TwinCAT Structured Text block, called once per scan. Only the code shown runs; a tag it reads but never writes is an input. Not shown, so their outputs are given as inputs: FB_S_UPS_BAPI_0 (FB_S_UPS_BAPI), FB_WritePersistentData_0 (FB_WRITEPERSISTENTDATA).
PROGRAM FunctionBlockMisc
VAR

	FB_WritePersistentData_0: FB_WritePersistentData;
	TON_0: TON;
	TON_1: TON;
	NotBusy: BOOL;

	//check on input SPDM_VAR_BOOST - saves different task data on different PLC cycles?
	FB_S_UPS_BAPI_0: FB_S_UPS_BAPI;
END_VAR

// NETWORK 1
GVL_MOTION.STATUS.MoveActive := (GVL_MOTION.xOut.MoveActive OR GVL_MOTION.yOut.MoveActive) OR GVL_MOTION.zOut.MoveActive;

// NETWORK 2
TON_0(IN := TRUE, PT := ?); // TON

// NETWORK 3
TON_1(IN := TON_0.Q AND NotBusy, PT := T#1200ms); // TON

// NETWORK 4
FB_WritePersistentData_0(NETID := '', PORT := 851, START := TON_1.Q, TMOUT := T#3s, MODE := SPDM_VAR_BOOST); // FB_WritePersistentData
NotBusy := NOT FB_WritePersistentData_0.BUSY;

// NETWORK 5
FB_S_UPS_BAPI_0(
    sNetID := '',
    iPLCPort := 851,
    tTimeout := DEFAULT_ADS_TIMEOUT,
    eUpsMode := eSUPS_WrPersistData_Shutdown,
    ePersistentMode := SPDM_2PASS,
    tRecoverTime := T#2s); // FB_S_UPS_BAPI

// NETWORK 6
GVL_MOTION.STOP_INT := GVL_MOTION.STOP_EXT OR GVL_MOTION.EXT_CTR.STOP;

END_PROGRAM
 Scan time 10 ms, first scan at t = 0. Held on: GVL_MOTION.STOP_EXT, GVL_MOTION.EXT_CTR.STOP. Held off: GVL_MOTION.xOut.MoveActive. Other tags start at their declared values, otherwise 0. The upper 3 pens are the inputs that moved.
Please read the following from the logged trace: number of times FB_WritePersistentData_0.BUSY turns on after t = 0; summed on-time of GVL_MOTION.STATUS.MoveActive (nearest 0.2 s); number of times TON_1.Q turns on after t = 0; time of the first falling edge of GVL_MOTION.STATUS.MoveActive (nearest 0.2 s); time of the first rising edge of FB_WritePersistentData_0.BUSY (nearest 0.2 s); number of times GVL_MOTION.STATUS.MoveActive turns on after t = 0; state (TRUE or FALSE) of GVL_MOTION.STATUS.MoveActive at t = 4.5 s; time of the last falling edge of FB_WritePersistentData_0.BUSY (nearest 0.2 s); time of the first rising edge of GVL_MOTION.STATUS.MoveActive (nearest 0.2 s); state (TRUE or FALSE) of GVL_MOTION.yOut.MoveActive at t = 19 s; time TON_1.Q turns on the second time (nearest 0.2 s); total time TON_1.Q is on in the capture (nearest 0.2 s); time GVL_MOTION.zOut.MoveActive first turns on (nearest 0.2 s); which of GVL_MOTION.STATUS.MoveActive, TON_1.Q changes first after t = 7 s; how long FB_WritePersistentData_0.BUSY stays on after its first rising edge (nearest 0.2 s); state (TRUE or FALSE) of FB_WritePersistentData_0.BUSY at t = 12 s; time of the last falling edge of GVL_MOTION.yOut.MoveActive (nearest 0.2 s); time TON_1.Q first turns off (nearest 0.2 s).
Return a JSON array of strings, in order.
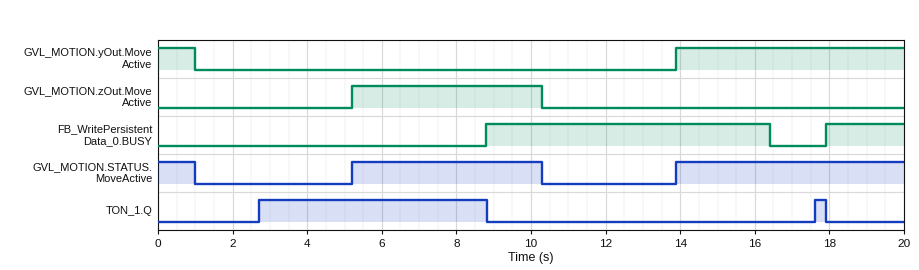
["2", "12.2 s", "2", "1.0 s", "8.8 s", "2", "FALSE", "16.4 s", "5.2 s", "TRUE", "17.6 s", "6.4 s", "5.2 s", "TON_1.Q", "7.6 s", "TRUE", "1.0 s", "8.8 s"]
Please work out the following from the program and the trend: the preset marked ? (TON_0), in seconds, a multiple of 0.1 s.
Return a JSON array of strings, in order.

["1.5 s"]
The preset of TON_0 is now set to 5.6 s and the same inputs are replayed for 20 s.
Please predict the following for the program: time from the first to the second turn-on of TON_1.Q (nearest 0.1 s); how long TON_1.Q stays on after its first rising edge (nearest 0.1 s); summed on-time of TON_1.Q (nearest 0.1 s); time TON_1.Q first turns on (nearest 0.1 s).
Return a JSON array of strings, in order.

["10.8 s", "2.0 s", "2.3 s", "6.8 s"]
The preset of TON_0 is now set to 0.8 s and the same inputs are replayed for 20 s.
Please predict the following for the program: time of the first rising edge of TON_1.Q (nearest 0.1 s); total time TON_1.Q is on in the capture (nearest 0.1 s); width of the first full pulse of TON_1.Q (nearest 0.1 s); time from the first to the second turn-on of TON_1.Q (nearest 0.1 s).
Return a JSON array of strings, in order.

["2.0 s", "7.1 s", "6.8 s", "15.6 s"]
